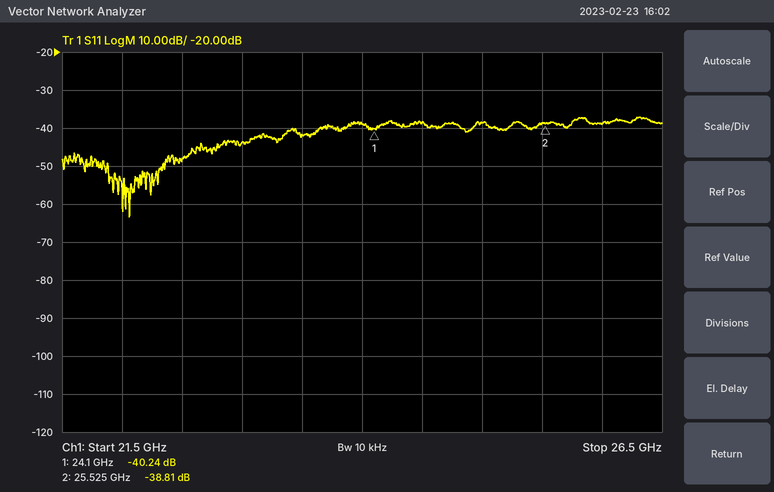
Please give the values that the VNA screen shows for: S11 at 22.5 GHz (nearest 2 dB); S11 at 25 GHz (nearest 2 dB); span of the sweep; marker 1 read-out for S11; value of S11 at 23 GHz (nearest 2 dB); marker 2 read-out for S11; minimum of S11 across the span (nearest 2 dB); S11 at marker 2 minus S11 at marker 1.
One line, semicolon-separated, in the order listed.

-48 dB; -38 dB; 5 GHz; -40.24 dB; -44 dB; -38.81 dB; -64 dB; 1.43 dB
